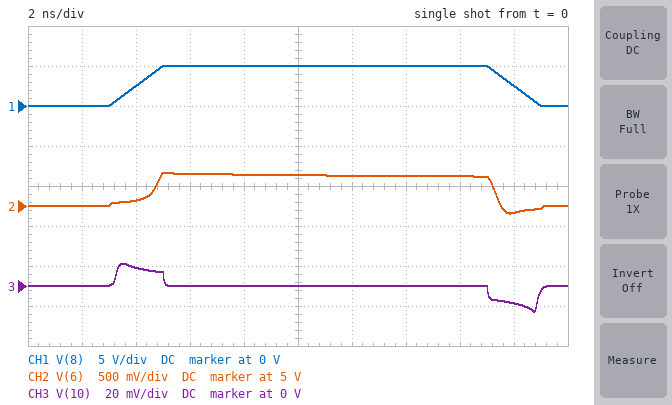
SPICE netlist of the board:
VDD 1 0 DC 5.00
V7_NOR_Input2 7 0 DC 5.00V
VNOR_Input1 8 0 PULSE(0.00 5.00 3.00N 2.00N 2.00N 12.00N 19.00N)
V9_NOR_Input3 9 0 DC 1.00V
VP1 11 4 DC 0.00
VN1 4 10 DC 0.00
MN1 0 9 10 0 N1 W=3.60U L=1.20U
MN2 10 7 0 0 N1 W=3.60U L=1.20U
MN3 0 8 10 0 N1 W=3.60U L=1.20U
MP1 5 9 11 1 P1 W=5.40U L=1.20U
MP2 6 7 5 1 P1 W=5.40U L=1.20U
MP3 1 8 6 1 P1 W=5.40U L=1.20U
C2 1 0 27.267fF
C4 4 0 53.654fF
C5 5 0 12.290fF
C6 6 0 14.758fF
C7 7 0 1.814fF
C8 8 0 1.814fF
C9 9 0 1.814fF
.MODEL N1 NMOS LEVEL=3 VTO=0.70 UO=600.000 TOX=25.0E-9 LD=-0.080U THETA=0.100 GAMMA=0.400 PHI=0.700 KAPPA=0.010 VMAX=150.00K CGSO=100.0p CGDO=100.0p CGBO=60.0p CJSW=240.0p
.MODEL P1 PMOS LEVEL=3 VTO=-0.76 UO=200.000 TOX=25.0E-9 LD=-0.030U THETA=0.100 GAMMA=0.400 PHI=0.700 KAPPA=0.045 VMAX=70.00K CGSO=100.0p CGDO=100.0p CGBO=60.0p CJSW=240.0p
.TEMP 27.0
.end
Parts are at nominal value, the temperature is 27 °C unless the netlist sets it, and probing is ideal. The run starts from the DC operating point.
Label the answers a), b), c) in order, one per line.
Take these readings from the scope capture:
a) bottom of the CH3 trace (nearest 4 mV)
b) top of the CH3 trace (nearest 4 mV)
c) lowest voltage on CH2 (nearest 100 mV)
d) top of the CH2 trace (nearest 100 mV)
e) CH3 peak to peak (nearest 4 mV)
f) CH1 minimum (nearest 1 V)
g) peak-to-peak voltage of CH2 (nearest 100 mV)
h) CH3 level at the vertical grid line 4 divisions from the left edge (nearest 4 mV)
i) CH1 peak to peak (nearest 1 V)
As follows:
a) -12 mV
b) 12 mV
c) 4.9 V
d) 5.4 V
e) 24 mV
f) 0 V
g) 500 mV
h) 0 V
i) 5 V
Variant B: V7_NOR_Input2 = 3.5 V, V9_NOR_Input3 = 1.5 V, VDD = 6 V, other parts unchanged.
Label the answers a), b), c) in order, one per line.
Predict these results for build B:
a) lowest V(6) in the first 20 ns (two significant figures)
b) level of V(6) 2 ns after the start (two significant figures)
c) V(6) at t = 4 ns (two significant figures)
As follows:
a) 4.7 V
b) 5.8 V
c) 5.7 V
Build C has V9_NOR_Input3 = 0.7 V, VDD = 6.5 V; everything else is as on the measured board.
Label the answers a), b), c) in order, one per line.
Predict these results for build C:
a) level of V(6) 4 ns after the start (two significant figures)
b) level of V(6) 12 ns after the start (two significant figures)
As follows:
a) 6.5 V
b) 6.3 V
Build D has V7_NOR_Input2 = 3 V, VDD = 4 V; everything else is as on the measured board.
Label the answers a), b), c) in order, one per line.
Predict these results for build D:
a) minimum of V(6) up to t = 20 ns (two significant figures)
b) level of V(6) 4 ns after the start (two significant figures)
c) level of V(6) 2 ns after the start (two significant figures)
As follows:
a) 3.8 V
b) 4.1 V
c) 4.0 V
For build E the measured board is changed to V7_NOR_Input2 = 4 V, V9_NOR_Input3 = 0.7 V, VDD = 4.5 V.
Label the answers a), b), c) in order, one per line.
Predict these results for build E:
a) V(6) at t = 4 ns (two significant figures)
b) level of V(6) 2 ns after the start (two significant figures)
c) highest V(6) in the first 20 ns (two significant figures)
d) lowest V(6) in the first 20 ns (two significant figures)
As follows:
a) 4.6 V
b) 4.5 V
c) 4.8 V
d) 4.4 V
